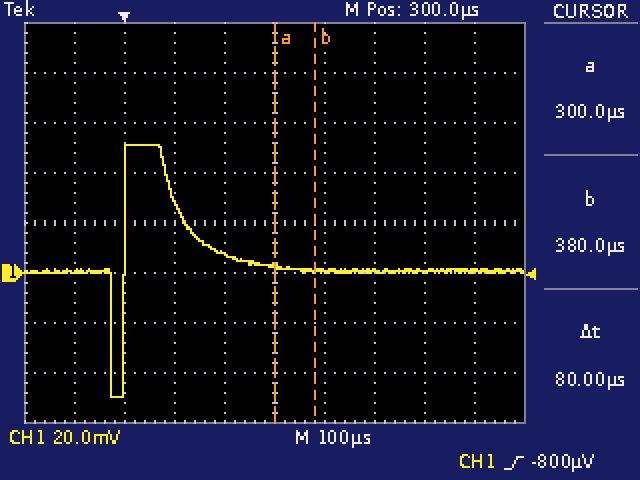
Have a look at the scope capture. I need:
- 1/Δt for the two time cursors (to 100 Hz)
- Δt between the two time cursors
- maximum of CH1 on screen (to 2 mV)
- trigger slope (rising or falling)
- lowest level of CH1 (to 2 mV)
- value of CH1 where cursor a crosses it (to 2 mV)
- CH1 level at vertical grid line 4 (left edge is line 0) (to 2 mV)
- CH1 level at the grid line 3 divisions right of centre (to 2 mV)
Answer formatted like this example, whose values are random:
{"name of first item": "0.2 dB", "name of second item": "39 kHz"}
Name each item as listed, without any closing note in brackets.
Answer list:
{"1/Δt for the two time cursors": "12.5 kHz", "Δt between the two time cursors": "80 µs", "maximum of CH1 on screen": "52 mV", "trigger slope": "rising", "lowest level of CH1": "-50 mV", "value of CH1 where cursor a crosses it": "2 mV", "CH1 level at vertical grid line 4 (left edge is line 0)": "8 mV", "CH1 level at the grid line 3 divisions right of centre": "0 mV"}
